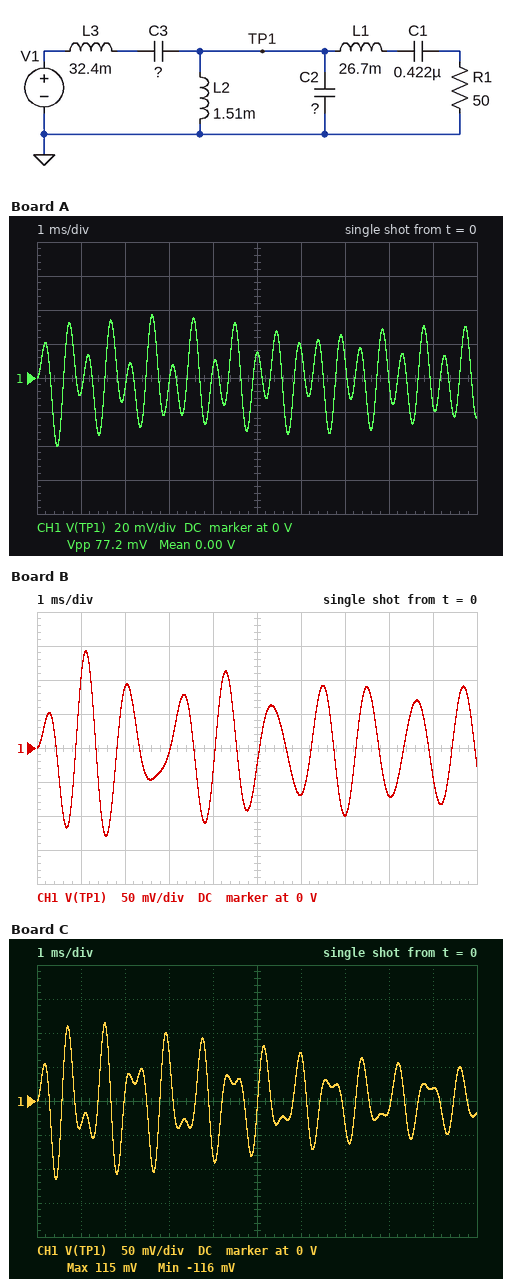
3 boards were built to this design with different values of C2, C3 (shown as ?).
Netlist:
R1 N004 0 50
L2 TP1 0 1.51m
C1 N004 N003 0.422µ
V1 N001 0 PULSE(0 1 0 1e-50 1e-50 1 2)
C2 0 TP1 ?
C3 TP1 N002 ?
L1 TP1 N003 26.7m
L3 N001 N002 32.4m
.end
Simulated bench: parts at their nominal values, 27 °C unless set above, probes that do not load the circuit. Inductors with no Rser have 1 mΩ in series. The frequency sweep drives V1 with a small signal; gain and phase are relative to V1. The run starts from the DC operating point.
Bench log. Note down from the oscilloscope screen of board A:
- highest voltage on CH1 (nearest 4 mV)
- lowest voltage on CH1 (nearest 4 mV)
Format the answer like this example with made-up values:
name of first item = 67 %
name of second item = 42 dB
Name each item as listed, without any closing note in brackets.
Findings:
highest voltage on CH1 = 36 mV
lowest voltage on CH1 = -40 mV
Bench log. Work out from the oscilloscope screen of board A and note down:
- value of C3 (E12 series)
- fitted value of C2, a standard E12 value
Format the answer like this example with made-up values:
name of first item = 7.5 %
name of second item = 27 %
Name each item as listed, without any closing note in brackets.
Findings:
value of C3 = 180 nF
fitted value of C2, a standard E12 value = 12 µF
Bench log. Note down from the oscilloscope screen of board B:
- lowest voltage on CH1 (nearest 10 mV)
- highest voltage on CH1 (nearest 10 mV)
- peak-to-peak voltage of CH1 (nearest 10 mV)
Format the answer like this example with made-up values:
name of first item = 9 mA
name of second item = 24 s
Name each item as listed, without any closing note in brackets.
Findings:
lowest voltage on CH1 = -130 mV
highest voltage on CH1 = 140 mV
peak-to-peak voltage of CH1 = 270 mV
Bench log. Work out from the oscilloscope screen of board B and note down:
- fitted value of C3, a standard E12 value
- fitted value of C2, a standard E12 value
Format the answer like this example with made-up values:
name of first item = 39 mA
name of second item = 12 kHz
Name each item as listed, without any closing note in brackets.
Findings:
fitted value of C3, a standard E12 value = 820 nF
fitted value of C2, a standard E12 value = 10 µF
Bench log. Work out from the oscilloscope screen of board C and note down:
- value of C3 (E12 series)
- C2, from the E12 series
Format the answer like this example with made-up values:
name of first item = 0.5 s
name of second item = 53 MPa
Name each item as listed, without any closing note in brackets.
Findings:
value of C3 = 390 nF
C2, from the E12 series = 3.9 µF
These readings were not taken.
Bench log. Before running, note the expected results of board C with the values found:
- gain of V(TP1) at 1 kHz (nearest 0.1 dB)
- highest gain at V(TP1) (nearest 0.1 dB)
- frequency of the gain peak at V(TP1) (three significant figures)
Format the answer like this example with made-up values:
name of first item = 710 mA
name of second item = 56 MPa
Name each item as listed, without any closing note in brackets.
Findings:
gain of V(TP1) at 1 kHz = -23.3 dB
highest gain at V(TP1) = 11.6 dB
frequency of the gain peak at V(TP1) = 1.35 kHz
